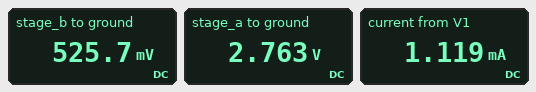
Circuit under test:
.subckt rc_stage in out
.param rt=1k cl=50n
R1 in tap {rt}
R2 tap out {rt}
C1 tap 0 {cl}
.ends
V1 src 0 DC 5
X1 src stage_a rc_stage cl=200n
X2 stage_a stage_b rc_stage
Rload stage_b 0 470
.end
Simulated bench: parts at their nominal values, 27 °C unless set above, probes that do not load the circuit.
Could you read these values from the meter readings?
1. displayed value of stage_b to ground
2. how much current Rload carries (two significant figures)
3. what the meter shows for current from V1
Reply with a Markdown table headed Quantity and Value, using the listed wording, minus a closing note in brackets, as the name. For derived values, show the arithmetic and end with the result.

| Quantity | Value |
|---|---|
| displayed value of stage_b to ground | 525.7 mV |
| how much current Rload carries | (525.7 mV) / 470 Ω = 1.1 mA |
| what the meter shows for current from V1 | 1.119 mA |
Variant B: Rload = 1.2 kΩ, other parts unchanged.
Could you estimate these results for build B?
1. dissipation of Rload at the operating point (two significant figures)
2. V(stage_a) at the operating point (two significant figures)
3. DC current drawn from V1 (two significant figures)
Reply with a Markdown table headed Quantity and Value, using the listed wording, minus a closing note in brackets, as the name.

| Quantity | Value |
|---|---|
| dissipation of Rload at the operating point | 1.1 mW |
| V(stage_a) at the operating point | 3.1 V |
| DC current drawn from V1 | 960 µA |
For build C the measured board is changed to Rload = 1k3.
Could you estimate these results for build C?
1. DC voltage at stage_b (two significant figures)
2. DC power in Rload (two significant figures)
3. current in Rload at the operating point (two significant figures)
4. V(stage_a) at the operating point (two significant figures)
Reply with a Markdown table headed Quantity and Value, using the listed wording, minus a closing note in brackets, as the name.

| Quantity | Value |
|---|---|
| DC voltage at stage_b | 1.2 V |
| DC power in Rload | 1.2 mW |
| current in Rload at the operating point | 940 µA |
| V(stage_a) at the operating point | 3.1 V |
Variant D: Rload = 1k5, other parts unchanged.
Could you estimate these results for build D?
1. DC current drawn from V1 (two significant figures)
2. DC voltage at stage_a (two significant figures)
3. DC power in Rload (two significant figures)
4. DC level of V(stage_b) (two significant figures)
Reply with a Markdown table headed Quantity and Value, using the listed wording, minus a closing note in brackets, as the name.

| Quantity | Value |
|---|---|
| DC current drawn from V1 | 910 µA |
| DC voltage at stage_a | 3.2 V |
| DC power in Rload | 1.2 mW |
| DC level of V(stage_b) | 1.4 V |
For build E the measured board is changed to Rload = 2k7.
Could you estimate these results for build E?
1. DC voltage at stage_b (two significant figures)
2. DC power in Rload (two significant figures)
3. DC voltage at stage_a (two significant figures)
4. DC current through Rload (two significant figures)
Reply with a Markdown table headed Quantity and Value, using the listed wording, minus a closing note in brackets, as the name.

| Quantity | Value |
|---|---|
| DC voltage at stage_b | 2.0 V |
| DC power in Rload | 1.5 mW |
| DC voltage at stage_a | 3.5 V |
| DC current through Rload | 750 µA |
